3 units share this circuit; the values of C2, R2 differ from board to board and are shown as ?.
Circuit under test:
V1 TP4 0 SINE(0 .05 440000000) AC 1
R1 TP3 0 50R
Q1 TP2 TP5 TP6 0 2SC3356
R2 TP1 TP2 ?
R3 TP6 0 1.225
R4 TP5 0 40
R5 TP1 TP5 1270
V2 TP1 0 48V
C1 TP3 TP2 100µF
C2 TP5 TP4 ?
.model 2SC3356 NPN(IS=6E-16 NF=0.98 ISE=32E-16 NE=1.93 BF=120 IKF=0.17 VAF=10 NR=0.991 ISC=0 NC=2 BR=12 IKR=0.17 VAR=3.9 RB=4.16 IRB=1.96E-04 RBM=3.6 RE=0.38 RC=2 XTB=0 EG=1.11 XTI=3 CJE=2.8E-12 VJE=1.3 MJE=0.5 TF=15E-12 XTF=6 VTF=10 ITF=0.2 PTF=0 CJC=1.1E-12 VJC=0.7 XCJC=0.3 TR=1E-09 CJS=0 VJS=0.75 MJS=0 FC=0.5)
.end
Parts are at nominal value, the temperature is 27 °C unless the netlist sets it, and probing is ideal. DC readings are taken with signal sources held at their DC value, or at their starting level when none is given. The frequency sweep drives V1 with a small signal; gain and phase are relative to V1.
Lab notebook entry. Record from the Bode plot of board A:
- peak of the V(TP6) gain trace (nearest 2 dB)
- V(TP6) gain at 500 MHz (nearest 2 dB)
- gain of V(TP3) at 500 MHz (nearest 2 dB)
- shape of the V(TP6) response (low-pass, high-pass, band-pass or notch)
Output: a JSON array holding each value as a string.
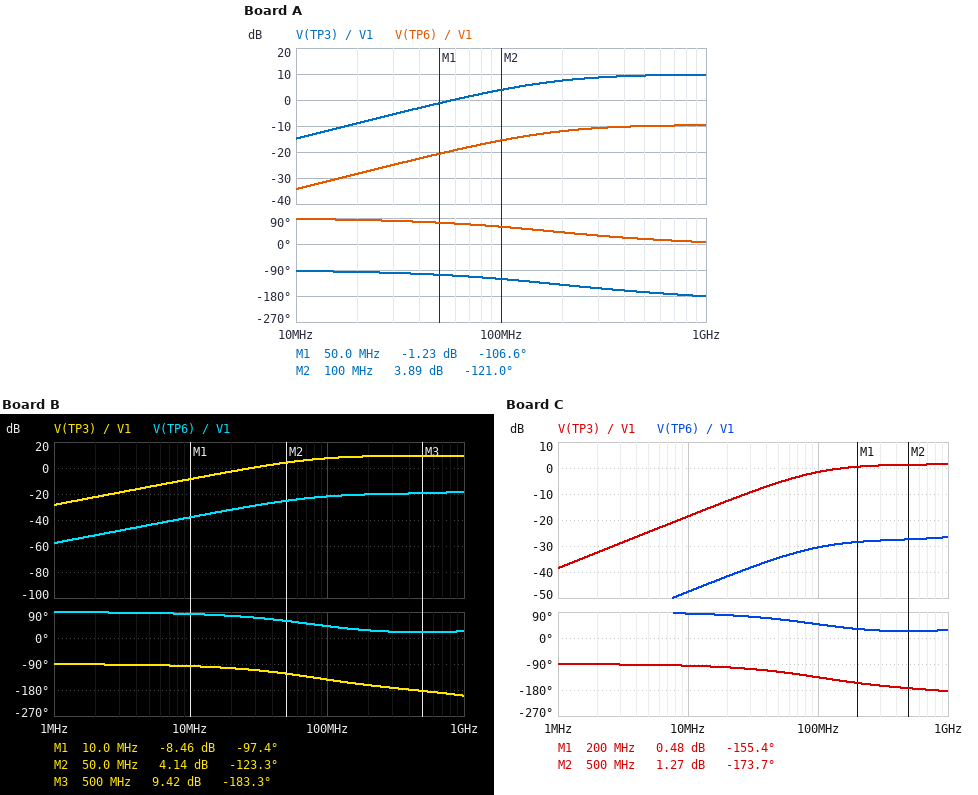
["-10 dB", "-10 dB", "10 dB", "high-pass"]
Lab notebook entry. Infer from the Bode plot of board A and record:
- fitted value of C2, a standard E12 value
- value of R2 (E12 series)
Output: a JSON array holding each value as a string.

["12 pF", "15 Ω"]
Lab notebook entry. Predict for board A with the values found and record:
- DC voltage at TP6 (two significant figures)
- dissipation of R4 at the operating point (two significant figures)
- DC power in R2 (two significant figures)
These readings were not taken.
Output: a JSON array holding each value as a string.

["450 mV", "51 mW", "2.0 W"]
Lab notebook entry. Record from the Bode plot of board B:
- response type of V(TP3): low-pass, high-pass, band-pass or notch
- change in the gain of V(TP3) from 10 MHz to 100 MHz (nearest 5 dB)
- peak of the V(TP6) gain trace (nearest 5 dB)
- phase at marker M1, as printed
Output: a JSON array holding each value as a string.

["high-pass", "15 dB", "-20 dB", "-97.4 deg"]
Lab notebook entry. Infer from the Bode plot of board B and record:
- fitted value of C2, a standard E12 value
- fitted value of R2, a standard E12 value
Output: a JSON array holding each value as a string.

["15 pF", "150 Ω"]
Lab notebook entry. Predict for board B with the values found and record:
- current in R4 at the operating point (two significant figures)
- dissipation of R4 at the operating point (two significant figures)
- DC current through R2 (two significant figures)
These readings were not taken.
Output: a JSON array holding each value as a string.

["33 mA", "44 mW", "270 mA"]
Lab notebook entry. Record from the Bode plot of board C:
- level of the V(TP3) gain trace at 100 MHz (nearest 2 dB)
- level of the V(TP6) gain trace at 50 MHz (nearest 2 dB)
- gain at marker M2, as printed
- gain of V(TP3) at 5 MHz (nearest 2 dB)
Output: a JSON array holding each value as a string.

["-2 dB", "-34 dB", "1.27 dB", "-24 dB"]
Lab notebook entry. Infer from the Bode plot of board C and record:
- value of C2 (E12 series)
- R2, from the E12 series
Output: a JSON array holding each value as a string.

["3.9 pF", "120 Ω"]
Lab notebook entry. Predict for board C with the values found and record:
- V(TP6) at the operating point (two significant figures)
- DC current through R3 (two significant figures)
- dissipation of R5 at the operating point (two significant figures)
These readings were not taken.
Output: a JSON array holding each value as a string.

["370 mV", "300 mA", "1.7 W"]
